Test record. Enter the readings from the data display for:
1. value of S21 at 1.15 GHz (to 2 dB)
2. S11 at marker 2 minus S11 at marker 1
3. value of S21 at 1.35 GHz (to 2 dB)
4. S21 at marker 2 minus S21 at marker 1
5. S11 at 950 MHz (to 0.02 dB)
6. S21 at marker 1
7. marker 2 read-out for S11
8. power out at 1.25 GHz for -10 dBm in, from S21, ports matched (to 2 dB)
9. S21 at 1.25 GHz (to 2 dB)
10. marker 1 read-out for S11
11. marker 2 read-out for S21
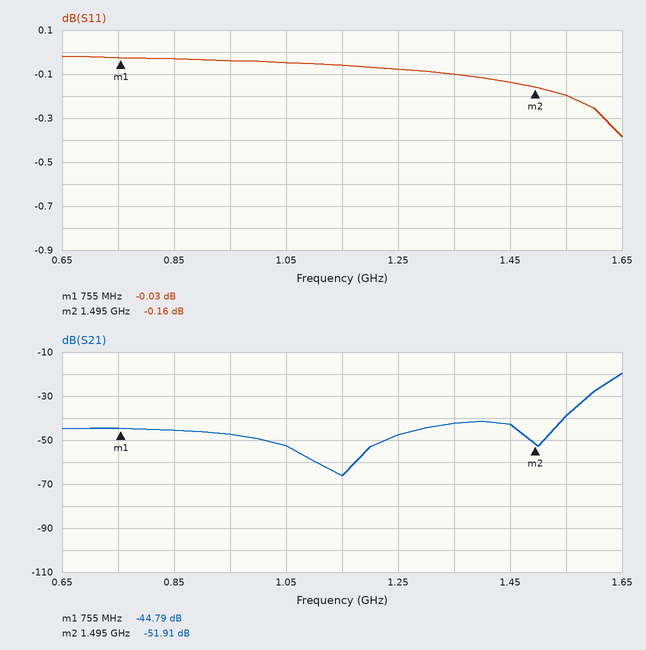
-66 dB
-0.13 dB
-42 dB
-7.12 dB
-0.04 dB
-44.79 dB
-0.16 dB
-58 dBm
-48 dB
-0.03 dB
-51.91 dB
